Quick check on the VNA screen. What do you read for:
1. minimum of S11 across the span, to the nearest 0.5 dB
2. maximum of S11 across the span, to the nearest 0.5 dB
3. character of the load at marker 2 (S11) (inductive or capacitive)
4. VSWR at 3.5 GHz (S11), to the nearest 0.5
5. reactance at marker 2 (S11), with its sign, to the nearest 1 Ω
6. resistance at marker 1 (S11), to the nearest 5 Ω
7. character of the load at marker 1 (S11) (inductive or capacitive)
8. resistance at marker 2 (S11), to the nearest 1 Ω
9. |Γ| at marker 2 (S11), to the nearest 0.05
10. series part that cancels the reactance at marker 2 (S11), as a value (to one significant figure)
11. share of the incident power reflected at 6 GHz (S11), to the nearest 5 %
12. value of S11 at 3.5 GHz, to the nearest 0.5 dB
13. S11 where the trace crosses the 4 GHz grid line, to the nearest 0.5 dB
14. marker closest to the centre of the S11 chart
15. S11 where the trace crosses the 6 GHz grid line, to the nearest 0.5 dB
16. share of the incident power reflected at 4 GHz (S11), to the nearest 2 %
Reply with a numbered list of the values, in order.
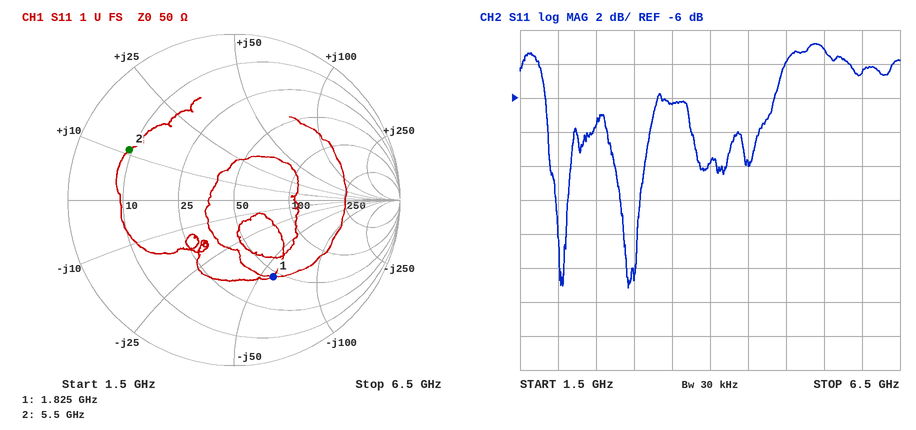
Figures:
1. -17.0 dB
2. -3.0 dB
3. inductive
4. 3.0
5. +11 Ω
6. 45 Ω
7. capacitive
8. 9 Ω
9. 0.70
10. 3 pF
11. 35 %
12. -6.5 dB
13. -10.0 dB
14. marker 1
15. -4.5 dB
16. 10 %
